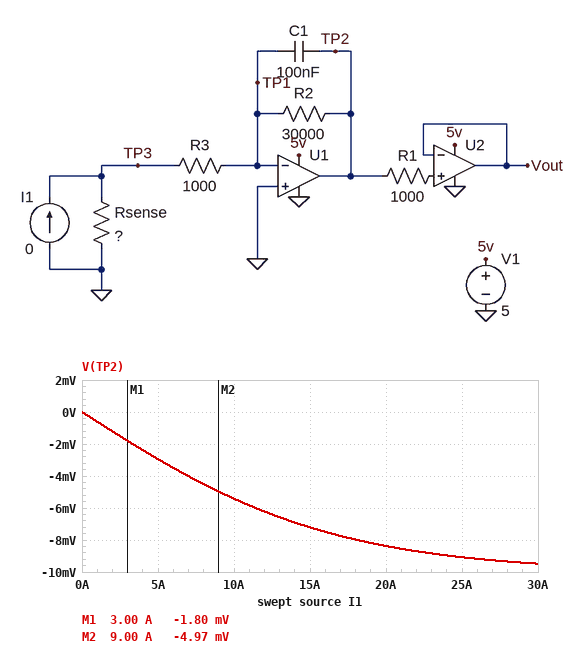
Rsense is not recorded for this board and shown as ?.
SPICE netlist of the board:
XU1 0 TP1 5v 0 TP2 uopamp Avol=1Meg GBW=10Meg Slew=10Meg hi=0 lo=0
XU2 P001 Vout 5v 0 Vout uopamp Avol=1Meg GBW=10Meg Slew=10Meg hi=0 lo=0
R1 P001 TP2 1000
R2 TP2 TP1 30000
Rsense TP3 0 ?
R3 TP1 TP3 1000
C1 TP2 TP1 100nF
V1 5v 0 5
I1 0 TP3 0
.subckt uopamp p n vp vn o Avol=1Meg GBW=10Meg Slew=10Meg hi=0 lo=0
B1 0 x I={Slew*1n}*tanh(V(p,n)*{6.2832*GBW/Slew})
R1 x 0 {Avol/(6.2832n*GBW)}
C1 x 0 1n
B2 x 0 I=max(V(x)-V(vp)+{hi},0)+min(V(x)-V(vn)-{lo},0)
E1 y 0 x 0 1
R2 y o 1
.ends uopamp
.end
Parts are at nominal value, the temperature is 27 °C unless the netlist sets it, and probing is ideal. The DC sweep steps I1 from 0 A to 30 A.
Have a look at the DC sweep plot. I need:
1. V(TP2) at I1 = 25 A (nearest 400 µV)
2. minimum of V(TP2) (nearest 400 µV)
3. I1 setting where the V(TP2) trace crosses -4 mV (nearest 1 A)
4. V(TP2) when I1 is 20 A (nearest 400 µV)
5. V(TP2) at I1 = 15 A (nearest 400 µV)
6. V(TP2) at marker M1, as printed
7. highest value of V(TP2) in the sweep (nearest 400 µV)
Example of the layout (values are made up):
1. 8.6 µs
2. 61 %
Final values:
1. -9.2 mV
2. -9.6 mV
3. 7 A
4. -8.4 mV
5. -7.2 mV
6. -1.80 mV
7. 0 V
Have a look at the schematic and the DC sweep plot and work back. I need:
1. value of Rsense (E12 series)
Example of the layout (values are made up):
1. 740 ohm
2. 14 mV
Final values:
1. 0.01 Ω
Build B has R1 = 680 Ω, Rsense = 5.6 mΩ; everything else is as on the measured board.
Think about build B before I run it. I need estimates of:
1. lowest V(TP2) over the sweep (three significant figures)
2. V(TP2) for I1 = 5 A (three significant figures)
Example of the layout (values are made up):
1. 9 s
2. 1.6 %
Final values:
1. -7.69 mV
2. -1.68 mV
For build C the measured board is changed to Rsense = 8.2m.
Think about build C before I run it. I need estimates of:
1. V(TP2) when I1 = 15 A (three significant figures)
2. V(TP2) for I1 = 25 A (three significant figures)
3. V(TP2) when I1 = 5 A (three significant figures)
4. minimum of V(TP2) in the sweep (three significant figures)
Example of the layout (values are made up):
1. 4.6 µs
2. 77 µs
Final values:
1. -6.33 mV
2. -8.46 mV
3. -2.44 mV
4. -9.03 mV
